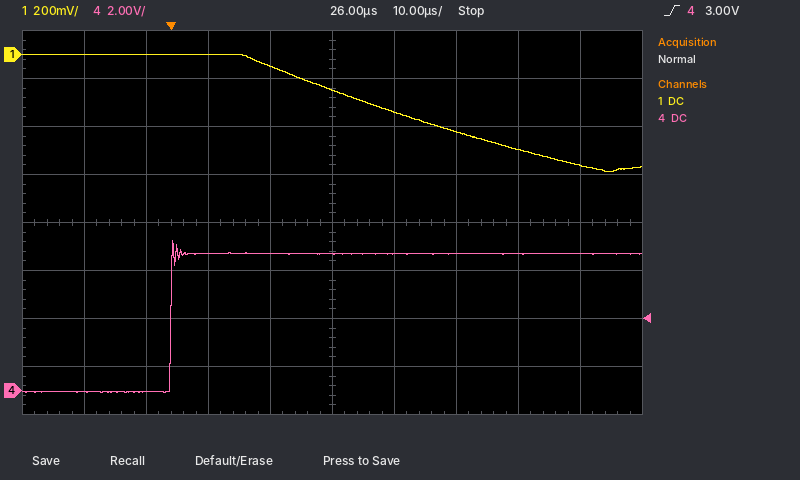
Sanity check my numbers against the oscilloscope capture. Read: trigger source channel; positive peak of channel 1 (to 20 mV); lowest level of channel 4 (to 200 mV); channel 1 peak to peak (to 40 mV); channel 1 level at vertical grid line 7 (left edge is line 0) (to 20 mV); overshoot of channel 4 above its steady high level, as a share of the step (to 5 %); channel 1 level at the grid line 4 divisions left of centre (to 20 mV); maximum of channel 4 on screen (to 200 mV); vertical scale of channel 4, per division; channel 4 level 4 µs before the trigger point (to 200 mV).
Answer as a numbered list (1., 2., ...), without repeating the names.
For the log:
1. channel 4
2. 0 mV
3. 0.0 V
4. 480 mV
5. -320 mV
6. 10 %
7. 0 mV
8. 6.2 V
9. 2 V
10. 0.0 V
